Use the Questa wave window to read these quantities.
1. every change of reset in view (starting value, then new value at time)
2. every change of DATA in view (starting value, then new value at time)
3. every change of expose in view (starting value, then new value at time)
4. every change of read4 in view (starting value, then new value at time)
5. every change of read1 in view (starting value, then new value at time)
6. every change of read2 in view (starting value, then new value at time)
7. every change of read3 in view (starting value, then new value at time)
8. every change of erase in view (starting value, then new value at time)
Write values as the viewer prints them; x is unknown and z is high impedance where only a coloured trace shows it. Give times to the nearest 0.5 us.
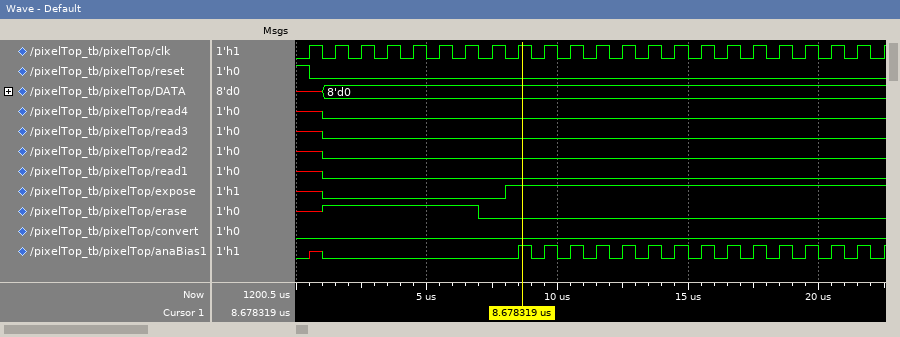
1, 0 at 0.5 us
x, 8'd0 at 1 us
x, 0 at 1 us, 1 at 8 us
x, 0 at 1 us
x, 0 at 1 us
x, 0 at 1 us
x, 0 at 1 us
x, 1 at 1 us, 0 at 7 us
